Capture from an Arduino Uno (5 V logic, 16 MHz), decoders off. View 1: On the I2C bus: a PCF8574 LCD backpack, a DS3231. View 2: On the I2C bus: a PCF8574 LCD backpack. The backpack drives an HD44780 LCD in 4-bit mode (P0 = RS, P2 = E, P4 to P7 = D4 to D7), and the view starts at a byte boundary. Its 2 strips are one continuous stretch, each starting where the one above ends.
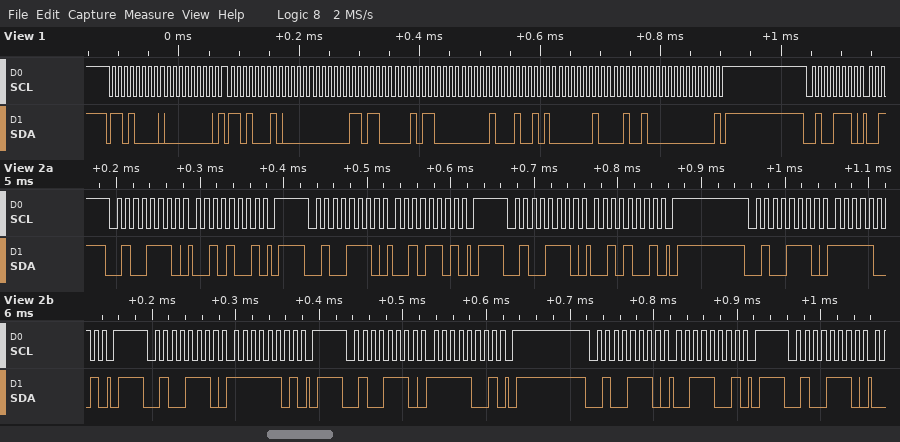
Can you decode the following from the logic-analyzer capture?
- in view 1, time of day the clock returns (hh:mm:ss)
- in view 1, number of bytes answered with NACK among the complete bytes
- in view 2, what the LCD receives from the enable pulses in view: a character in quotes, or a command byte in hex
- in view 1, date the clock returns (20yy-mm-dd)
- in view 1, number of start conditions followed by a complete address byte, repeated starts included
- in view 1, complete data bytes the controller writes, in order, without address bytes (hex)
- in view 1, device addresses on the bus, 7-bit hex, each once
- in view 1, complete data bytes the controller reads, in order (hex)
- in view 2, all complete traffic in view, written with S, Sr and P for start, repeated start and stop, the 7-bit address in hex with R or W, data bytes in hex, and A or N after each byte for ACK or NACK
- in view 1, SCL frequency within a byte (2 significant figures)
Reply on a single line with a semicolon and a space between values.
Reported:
16:36:00; 1; '/'; 2024-02-25; 3; 00; 0x68 0x27; 00 36 16 01 25 02 24 00; S 27W A 29 A P S 27W A 2D A P S 27W A 29 A P S 27W A F9 A P S 27W A FD A P S 27W A F9 A P S 27W A 39 A P S 27W A; 100 kHz
